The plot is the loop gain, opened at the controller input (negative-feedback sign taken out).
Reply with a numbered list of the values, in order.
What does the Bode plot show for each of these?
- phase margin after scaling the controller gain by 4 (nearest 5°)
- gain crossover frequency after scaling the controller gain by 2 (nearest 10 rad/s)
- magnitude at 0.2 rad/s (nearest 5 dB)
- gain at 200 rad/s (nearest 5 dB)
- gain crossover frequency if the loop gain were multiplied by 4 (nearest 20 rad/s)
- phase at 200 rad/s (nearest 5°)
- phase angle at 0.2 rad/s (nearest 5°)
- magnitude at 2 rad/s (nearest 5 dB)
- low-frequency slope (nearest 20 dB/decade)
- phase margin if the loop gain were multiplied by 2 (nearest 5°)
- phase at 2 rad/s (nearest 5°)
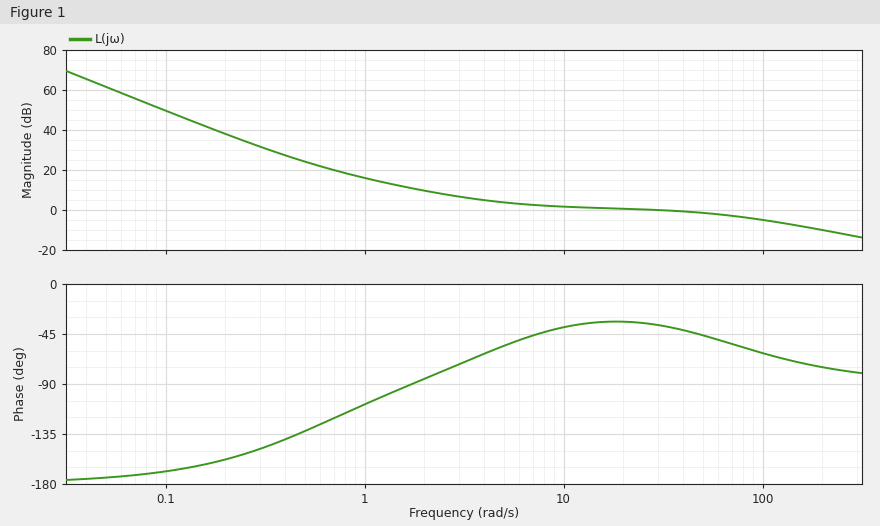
1. 100°
2. 120 rad/s
3. 40 dB
4. -10 dB
5. 260 rad/s
6. -75°
7. -160°
8. 10 dB
9. -40 dB/decade
10. 115°
11. -85°
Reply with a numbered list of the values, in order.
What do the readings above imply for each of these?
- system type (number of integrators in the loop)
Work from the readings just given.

1. 2
